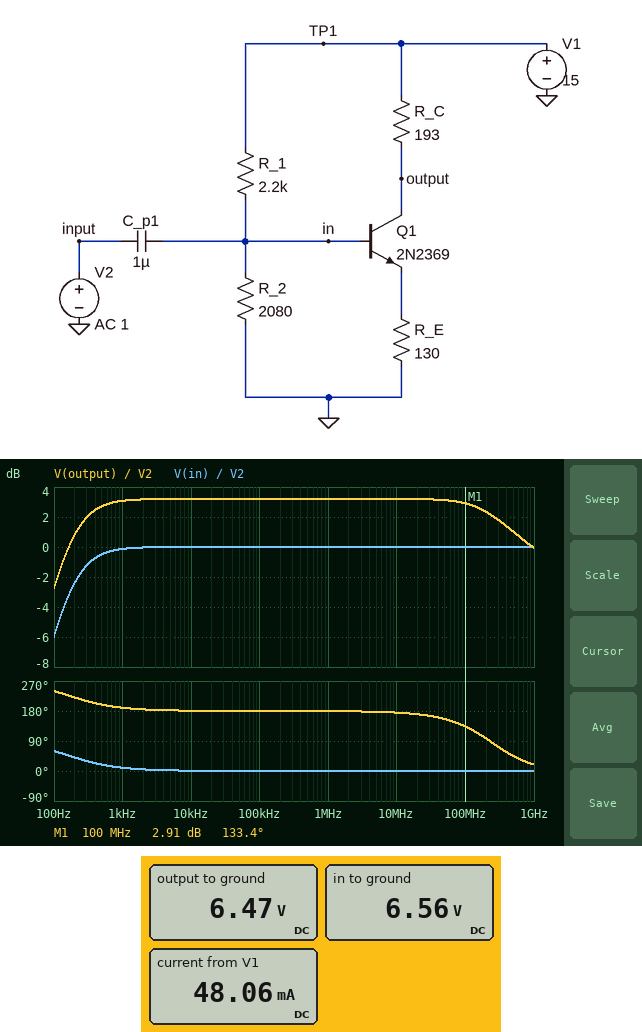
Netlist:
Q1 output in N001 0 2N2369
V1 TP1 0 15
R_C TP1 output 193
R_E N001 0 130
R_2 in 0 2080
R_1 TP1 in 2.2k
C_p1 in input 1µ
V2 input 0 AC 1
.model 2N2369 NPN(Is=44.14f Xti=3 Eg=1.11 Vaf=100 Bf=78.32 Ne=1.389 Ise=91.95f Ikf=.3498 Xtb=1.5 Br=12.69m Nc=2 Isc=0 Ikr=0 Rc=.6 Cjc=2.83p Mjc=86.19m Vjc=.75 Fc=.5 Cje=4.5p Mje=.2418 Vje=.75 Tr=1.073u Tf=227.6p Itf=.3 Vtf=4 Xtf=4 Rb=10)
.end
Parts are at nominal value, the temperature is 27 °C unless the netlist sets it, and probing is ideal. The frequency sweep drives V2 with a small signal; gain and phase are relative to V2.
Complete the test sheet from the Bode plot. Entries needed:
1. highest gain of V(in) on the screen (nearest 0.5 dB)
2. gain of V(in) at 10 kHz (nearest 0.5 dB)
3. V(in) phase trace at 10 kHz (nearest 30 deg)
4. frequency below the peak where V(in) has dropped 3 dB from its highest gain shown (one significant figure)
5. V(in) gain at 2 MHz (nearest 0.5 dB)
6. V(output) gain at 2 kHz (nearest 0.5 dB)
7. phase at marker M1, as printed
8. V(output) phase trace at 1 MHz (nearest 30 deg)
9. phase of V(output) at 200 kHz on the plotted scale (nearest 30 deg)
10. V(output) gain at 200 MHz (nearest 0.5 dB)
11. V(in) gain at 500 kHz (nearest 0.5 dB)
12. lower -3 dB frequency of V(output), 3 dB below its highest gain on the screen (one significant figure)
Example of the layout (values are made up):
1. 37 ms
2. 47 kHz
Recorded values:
1. 0 dB
2. 0 dB
3. 0 deg
4. 200 Hz
5. 0 dB
6. 3.0 dB
7. 133.4 deg
8. 180 deg
9. 180 deg
10. 2.5 dB
11. 0 dB
12. 200 Hz
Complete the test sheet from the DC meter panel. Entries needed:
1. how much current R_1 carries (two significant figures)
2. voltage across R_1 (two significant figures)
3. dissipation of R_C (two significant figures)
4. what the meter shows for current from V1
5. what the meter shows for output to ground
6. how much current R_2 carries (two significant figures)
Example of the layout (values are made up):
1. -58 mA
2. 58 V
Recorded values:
1. 3.8 mA
2. 8.4 V
3. 380 mW
4. 48.06 mA
5. 6.47 V
6. 3.2 mA
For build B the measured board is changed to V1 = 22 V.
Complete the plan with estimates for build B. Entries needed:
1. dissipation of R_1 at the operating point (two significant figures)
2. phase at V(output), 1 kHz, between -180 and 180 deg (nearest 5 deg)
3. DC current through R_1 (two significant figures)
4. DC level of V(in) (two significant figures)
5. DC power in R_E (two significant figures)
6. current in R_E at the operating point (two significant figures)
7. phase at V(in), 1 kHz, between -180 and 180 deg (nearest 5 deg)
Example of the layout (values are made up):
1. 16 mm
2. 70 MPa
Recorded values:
1. 71 mW
2. -160 deg
3. 5.7 mA
4. 9.5 V
5. 590 mW
6. 68 mA
7. 20 deg
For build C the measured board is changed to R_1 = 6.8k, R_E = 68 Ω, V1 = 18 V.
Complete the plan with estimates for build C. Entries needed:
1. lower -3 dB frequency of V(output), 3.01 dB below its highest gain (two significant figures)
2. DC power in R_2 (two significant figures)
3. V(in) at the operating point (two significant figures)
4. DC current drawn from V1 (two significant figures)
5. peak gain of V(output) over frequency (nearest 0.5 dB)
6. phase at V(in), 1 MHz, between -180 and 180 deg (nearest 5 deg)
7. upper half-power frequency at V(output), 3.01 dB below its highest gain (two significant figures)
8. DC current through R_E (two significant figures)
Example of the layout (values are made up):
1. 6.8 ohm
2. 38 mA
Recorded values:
1. 140 Hz
2. 5.4 mW
3. 3.4 V
4. 40 mA
5. 9.0 dB
6. 0 deg
7. 320 MHz
8. 39 mA
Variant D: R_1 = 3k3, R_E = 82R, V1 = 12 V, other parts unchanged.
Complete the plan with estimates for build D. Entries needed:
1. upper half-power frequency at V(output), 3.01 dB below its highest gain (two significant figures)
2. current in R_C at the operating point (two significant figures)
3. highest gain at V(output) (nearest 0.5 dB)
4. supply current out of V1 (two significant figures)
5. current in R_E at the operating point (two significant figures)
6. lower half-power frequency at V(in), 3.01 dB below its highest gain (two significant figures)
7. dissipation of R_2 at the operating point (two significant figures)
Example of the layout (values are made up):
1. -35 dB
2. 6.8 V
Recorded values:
1. 320 MHz
2. 38 mA
3. 7.0 dB
4. 41 mA
5. 39 mA
6. 160 Hz
7. 7.3 mW
